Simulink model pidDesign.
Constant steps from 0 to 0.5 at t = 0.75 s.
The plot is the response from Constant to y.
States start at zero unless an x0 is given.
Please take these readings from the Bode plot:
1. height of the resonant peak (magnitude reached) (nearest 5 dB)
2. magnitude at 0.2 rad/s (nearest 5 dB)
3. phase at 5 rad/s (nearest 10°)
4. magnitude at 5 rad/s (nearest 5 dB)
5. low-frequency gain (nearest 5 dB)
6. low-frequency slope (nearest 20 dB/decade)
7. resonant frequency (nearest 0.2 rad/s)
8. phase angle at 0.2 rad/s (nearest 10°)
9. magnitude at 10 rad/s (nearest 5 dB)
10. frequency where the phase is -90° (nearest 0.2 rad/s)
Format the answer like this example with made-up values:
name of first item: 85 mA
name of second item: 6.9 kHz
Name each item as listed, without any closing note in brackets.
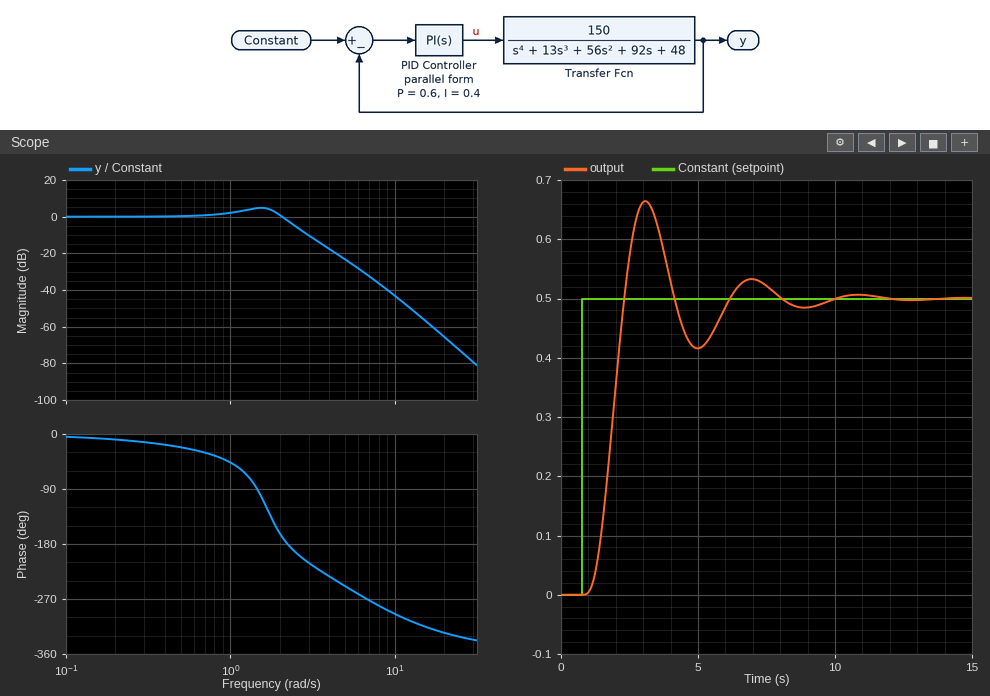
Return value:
height of the resonant peak (magnitude reached): 5 dB
magnitude at 0.2 rad/s: 0 dB
phase at 5 rad/s: -250°
magnitude at 5 rad/s: -25 dB
low-frequency gain: 0 dB
low-frequency slope: 0 dB/decade
resonant frequency: 1.6 rad/s
phase angle at 0.2 rad/s: -10°
magnitude at 10 rad/s: -45 dB
frequency where the phase is -90°: 1.4 rad/s
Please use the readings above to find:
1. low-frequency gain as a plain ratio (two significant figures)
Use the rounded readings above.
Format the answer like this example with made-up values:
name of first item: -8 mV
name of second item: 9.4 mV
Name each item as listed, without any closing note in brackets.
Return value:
low-frequency gain as a plain ratio: 1.0
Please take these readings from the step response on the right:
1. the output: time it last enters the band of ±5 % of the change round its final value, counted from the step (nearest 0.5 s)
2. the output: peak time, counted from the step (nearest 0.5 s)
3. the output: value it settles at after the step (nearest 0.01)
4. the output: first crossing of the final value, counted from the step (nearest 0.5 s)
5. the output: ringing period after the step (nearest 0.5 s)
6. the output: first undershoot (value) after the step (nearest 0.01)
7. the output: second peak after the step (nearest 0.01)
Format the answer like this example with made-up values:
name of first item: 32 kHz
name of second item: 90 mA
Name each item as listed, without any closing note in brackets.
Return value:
the output: time it last enters the band of ±5 % of the change round its final value, counted from the step: 6.5 s
the output: peak time, counted from the step: 2.5 s
the output: value it settles at after the step: 0.50
the output: first crossing of the final value, counted from the step: 1.5 s
the output: ringing period after the step: 4.0 s
the output: first undershoot (value) after the step: 0.42
the output: second peak after the step: 0.53
